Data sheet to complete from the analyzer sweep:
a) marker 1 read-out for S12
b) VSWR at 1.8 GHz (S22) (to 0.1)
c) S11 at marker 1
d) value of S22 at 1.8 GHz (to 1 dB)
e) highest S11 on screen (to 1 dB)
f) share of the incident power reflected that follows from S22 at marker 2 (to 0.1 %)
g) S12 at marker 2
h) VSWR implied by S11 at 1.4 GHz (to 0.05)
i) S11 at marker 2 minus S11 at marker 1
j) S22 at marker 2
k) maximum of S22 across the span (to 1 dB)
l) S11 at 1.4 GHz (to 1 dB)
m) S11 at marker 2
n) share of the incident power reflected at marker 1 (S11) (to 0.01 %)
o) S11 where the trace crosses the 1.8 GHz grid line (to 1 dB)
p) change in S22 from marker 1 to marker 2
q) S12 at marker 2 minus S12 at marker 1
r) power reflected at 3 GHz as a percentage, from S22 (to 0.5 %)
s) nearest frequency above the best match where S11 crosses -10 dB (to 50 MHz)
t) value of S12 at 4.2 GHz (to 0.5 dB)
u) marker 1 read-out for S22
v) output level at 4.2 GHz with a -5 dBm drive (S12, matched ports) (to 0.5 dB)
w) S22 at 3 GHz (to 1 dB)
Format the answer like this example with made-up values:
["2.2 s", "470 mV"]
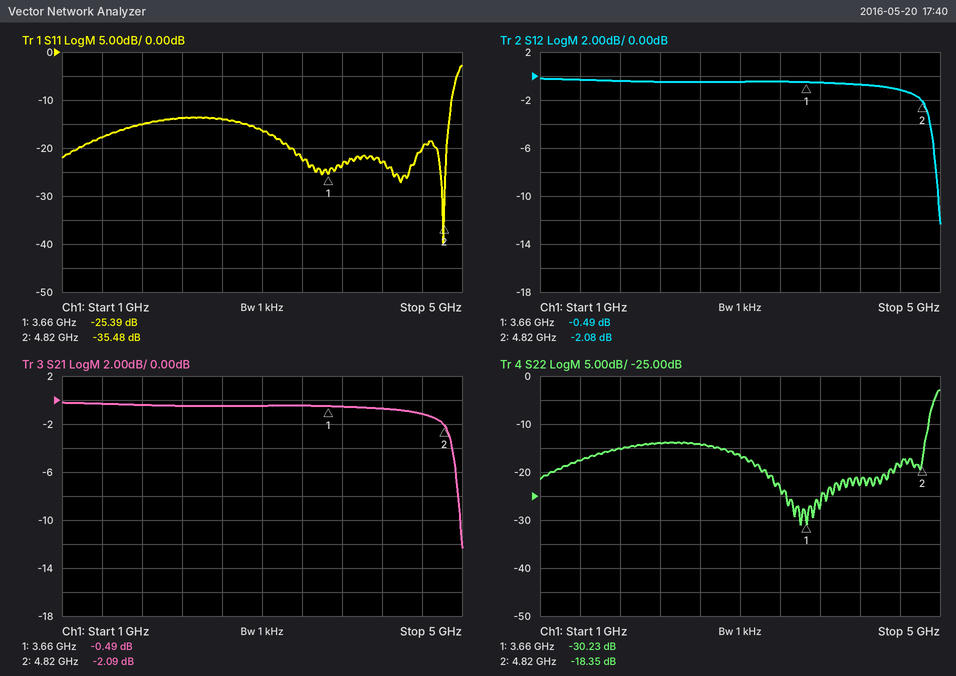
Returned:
["-0.49 dB", "1.4", "-25.39 dB", "-15 dB", "-3 dB", "1.5 %", "-2.08 dB", "1.30", "-10.09 dB", "-18.35 dB", "-3 dB", "-18 dB", "-35.48 dB", "0.29 %", "-15 dB", "11.88 dB", "-1.59 dB", "2.0 %", "4.90 GHz", "-0.5 dB", "-30.23 dB", "-5.5 dBm", "-17 dB"]
